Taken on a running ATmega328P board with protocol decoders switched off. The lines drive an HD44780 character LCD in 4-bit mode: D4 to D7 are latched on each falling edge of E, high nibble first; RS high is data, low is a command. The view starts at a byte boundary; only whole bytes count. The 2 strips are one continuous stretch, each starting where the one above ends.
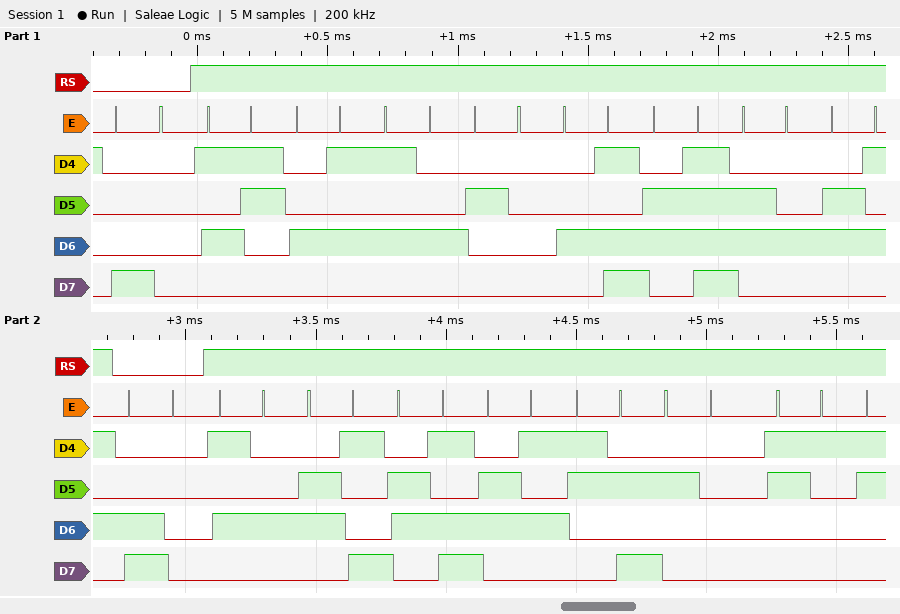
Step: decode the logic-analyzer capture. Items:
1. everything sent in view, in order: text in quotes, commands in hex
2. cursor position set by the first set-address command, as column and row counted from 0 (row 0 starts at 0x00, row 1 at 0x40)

0x80 "SET Mode" 0xC0 "Time: 1"
column 0, row 0
